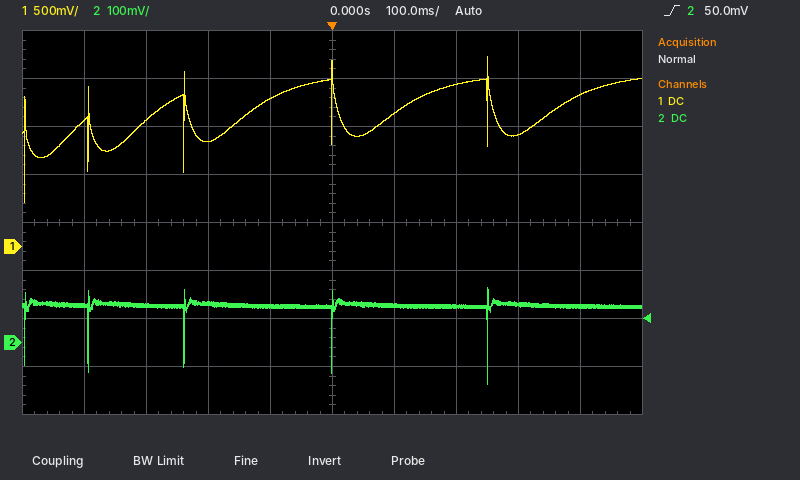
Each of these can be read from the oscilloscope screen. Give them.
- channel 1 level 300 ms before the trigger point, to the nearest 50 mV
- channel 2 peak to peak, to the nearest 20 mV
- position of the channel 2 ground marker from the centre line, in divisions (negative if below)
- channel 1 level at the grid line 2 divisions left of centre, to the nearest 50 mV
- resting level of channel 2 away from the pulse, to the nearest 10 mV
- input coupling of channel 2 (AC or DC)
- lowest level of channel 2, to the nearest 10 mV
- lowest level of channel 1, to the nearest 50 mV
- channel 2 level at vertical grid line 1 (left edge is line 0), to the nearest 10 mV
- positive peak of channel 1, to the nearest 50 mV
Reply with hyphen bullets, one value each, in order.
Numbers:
- 1.30 V
- 200 mV
- -2.5 div
- 1.10 V
- 80 mV
- DC
- -90 mV
- 450 mV
- 80 mV
- 2.00 V
